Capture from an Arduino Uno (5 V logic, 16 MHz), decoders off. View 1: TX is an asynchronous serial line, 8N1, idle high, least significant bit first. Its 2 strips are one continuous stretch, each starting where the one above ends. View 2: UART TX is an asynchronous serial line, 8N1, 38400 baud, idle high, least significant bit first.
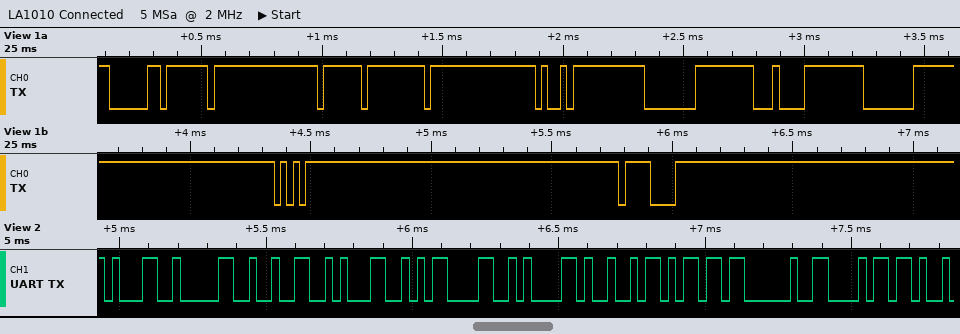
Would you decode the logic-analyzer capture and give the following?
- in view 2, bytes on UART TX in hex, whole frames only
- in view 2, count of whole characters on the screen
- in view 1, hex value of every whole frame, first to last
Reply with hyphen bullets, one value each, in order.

- 31 30 32 31 0D 0A 49 6D 20 68
- 10
- 60 FF BF FF E9 80 84 80 F5 0F
